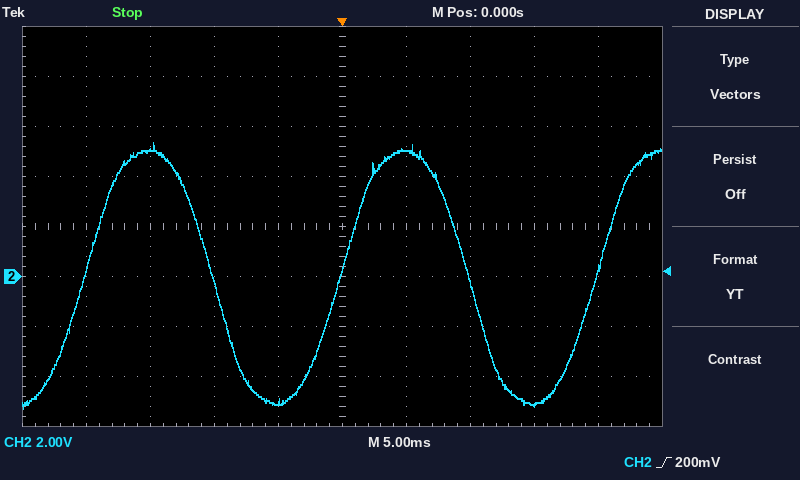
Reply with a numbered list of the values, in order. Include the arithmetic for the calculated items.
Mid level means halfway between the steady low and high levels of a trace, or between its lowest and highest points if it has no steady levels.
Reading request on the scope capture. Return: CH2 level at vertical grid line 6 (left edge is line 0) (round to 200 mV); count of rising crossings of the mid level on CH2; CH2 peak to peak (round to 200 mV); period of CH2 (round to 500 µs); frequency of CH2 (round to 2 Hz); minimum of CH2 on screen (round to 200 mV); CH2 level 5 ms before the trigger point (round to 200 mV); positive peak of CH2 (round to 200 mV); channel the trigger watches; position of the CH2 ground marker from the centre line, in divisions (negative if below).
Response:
1. 5.0 V
2. 3
3. 5.4 V − (-5.2 V) = 10.6 V
4. 20.0 ms
5. 1 / 20.0 ms ≈ 50 Hz
6. -5.2 V
7. -5.0 V
8. 5.4 V
9. CH2
10. -1.0 div
